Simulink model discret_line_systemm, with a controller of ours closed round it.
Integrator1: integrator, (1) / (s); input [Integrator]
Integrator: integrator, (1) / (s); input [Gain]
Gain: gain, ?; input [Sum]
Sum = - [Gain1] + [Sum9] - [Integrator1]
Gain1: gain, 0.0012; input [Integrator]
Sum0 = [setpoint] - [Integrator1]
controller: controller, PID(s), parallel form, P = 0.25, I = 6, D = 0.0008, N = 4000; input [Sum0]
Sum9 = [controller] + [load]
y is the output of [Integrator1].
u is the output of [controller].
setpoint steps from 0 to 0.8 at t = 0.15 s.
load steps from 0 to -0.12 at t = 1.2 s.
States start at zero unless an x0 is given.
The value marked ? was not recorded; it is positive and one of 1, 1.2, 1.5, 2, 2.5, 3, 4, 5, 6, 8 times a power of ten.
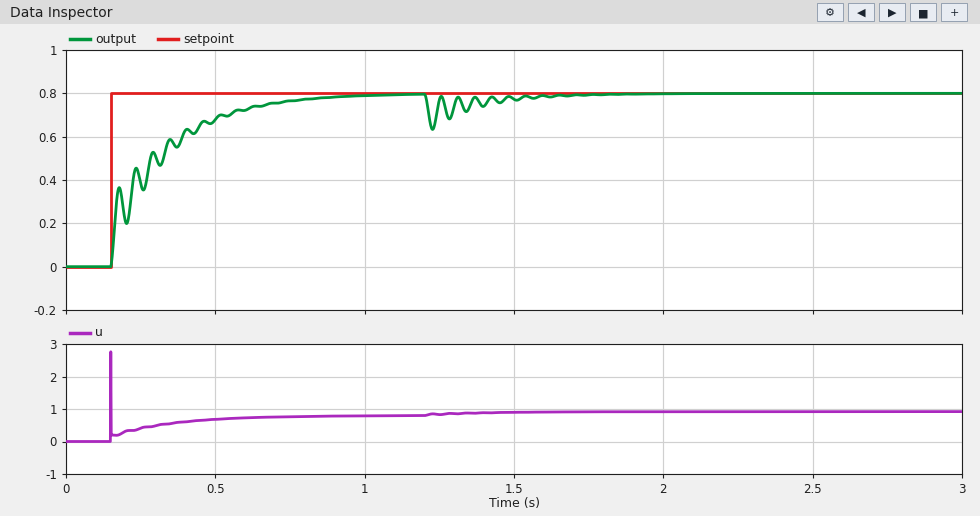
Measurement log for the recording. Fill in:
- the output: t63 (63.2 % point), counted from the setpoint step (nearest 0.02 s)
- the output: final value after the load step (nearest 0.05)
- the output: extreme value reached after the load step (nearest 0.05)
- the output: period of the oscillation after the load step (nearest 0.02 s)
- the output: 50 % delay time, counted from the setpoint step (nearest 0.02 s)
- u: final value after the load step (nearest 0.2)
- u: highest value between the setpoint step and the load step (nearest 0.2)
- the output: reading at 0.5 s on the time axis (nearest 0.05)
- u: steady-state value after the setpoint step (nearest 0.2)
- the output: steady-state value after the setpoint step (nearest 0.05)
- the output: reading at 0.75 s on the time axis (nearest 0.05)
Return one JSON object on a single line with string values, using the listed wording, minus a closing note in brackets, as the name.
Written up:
{"the output: t63 (63.2 % point), counted from the setpoint step": "0.14 s", "the output: final value after the load step": "0.80", "the output: extreme value reached after the load step": "0.65", "the output: period of the oscillation after the load step": "0.06 s", "the output: 50 % delay time, counted from the setpoint step": "0.08 s", "u: final value after the load step": "1.0", "u: highest value between the setpoint step and the load step": "2.8", "the output: reading at 0.5 s on the time axis": "0.70", "u: steady-state value after the setpoint step": "0.8", "the output: steady-state value after the setpoint step": "0.80", "the output: reading at 0.75 s on the time axis": "0.75"}
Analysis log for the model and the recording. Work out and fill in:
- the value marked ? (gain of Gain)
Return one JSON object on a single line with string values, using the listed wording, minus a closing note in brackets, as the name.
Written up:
{"the value marked ?": "10000"}
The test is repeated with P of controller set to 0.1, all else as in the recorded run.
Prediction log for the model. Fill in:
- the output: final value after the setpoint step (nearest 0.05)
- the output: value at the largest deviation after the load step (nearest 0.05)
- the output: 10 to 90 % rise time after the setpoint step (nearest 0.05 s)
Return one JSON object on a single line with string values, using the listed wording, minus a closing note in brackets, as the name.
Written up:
{"the output: final value after the setpoint step": "0.80", "the output: value at the largest deviation after the load step": "0.60", "the output: 10 to 90 % rise time after the setpoint step": "0.40 s"}
